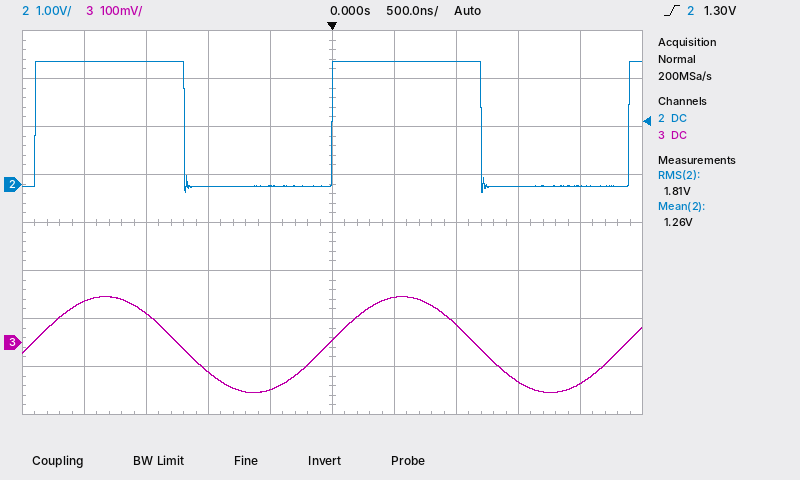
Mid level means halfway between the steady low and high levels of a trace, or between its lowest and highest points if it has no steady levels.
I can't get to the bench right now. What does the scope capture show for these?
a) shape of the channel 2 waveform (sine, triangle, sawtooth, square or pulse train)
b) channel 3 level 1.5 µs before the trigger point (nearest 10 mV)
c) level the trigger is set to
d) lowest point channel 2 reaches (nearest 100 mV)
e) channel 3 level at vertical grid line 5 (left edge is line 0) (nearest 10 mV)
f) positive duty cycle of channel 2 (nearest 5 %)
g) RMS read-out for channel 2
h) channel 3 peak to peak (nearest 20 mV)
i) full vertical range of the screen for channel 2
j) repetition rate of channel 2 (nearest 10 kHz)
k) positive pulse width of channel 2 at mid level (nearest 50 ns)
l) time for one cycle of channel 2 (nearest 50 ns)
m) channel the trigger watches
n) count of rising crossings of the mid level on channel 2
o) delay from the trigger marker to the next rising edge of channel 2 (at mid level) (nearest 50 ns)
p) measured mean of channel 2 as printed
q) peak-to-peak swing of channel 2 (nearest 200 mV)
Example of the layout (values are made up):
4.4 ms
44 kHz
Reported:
square
60 mV
1.30 V
-200 mV
0 mV
50 %
1.81 V
200 mV
8 V
420 kHz
1.20 µs
2.40 µs
channel 2
3
2.40 µs
1.26 V
2.8 V
